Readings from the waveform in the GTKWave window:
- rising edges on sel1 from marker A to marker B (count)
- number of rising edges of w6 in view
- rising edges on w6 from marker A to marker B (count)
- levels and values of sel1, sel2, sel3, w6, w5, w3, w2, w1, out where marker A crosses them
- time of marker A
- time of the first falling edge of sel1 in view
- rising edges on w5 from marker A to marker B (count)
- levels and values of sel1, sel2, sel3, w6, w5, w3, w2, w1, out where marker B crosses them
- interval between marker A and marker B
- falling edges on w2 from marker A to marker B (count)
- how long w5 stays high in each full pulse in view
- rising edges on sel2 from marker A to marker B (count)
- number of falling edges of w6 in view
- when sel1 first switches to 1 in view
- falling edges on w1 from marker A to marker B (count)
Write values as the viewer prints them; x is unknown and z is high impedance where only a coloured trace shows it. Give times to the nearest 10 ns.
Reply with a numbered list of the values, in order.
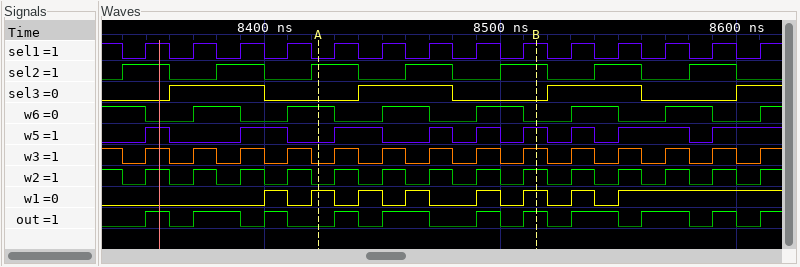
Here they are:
1. 5
2. 7
3. 2
4. sel1=0, sel2=1, sel3=0, w6=1, w5=0, w3=0, w2=0, w1=1, out=0
5. 8420 ns
6. 8340 ns
7. 4
8. sel1=1, sel2=1, sel3=0, w6=0, w5=1, w3=1, w2=1, w1=1, out=1
9. 90 ns
10. 4
11. 10 ns, 20 ns, 20 ns, 10 ns, 10 ns, 10 ns, 10 ns, 30 ns
12. 2
13. 7
14. 8350 ns
15. 4
